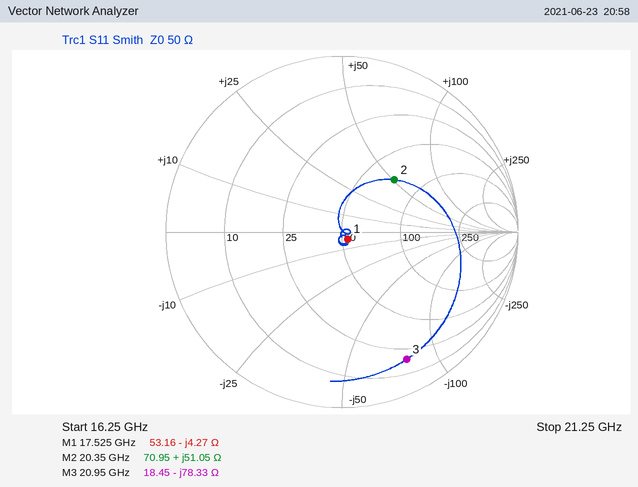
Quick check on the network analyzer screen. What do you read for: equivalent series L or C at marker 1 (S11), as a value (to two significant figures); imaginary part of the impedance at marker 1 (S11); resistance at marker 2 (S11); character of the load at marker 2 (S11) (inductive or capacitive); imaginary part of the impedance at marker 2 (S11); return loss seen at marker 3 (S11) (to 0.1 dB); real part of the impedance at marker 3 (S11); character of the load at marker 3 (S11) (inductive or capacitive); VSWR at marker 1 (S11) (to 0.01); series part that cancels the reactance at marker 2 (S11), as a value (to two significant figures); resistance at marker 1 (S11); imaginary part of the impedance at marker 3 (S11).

2.1 pF
-4.27 Ω
70.95 Ω
inductive
+51.05 Ω
1.8 dB
18.45 Ω
capacitive
1.11
150 fF
53.16 Ω
-78.33 Ω
